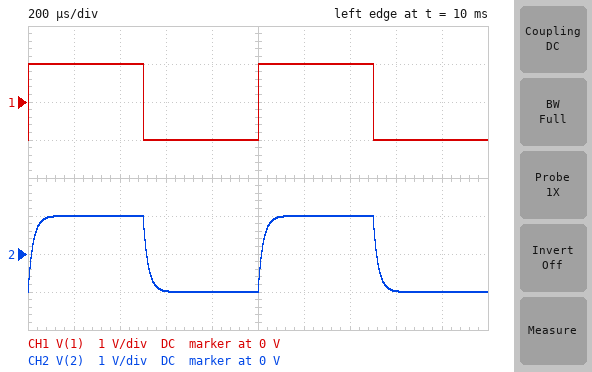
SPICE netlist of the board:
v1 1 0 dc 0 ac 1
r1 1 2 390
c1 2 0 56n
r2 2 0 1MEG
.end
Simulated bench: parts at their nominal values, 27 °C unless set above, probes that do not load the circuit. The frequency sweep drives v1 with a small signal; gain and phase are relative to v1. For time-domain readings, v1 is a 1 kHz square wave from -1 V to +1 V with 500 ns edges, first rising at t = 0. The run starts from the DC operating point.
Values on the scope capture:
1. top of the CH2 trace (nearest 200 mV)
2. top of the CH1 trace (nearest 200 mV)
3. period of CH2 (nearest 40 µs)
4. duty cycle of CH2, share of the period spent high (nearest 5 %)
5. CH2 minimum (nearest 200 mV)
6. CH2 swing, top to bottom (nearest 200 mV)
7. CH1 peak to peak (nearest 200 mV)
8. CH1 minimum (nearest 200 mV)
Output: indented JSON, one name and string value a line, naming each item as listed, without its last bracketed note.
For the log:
{
  "top of the CH2 trace": "1.0 V",
  "top of the CH1 trace": "1.0 V",
  "period of CH2": "1.00 ms",
  "duty cycle of CH2, share of the period spent high": "50 %",
  "CH2 minimum": "-1.0 V",
  "CH2 swing, top to bottom": "2.0 V",
  "CH1 peak to peak": "2.0 V",
  "CH1 minimum": "-1.0 V"
}
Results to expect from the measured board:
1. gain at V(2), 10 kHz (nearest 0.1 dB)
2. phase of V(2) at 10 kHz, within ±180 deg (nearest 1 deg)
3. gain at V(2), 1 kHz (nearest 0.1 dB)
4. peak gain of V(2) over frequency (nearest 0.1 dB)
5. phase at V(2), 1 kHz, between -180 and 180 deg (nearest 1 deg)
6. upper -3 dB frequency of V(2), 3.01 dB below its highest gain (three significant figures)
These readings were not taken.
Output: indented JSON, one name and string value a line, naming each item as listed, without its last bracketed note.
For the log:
{
  "gain at V(2), 10 kHz": "-4.6 dB",
  "phase of V(2) at 10 kHz, within ±180 deg": "-54 deg",
  "gain at V(2), 1 kHz": "-0.1 dB",
  "peak gain of V(2) over frequency": "0 dB",
  "phase at V(2), 1 kHz, between -180 and 180 deg": "-8 deg",
  "upper -3 dB frequency of V(2), 3.01 dB below its highest gain": "7.29 kHz"
}
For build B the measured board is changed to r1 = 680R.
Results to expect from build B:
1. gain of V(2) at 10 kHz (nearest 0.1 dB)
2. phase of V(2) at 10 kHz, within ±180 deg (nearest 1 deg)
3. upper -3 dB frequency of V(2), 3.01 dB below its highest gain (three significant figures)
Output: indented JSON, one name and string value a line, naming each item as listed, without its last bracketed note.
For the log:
{
  "gain of V(2) at 10 kHz": "-8.3 dB",
  "phase of V(2) at 10 kHz, within ±180 deg": "-67 deg",
  "upper -3 dB frequency of V(2), 3.01 dB below its highest gain": "4.18 kHz"
}
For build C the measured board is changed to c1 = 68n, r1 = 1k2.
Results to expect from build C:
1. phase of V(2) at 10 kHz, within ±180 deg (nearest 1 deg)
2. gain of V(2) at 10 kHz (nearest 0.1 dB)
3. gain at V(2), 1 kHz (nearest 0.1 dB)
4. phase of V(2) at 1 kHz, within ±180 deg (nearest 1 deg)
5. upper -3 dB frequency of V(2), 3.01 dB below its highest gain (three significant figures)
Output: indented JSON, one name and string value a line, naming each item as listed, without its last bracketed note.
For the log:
{
  "phase of V(2) at 10 kHz, within ±180 deg": "-79 deg",
  "gain of V(2) at 10 kHz": "-14.4 dB",
  "gain at V(2), 1 kHz": "-1.0 dB",
  "phase of V(2) at 1 kHz, within ±180 deg": "-27 deg",
  "upper -3 dB frequency of V(2), 3.01 dB below its highest gain": "1.95 kHz"
}
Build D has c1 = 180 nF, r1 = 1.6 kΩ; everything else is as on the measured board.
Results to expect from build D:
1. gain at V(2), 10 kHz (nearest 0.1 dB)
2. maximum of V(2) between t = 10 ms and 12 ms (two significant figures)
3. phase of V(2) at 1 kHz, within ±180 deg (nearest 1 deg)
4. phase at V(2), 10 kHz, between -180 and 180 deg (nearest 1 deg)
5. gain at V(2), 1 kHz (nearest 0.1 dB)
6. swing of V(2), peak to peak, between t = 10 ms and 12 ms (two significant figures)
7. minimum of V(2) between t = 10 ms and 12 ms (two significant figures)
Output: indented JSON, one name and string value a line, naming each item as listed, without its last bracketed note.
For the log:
{
  "gain at V(2), 10 kHz": "-25.2 dB",
  "maximum of V(2) between t = 10 ms and 12 ms": "700 mV",
  "phase of V(2) at 1 kHz, within ±180 deg": "-61 deg",
  "phase at V(2), 10 kHz, between -180 and 180 deg": "-87 deg",
  "gain at V(2), 1 kHz": "-6.3 dB",
  "swing of V(2), peak to peak, between t = 10 ms and 12 ms": "1.4 V",
  "minimum of V(2) between t = 10 ms and 12 ms": "-700 mV"
}
